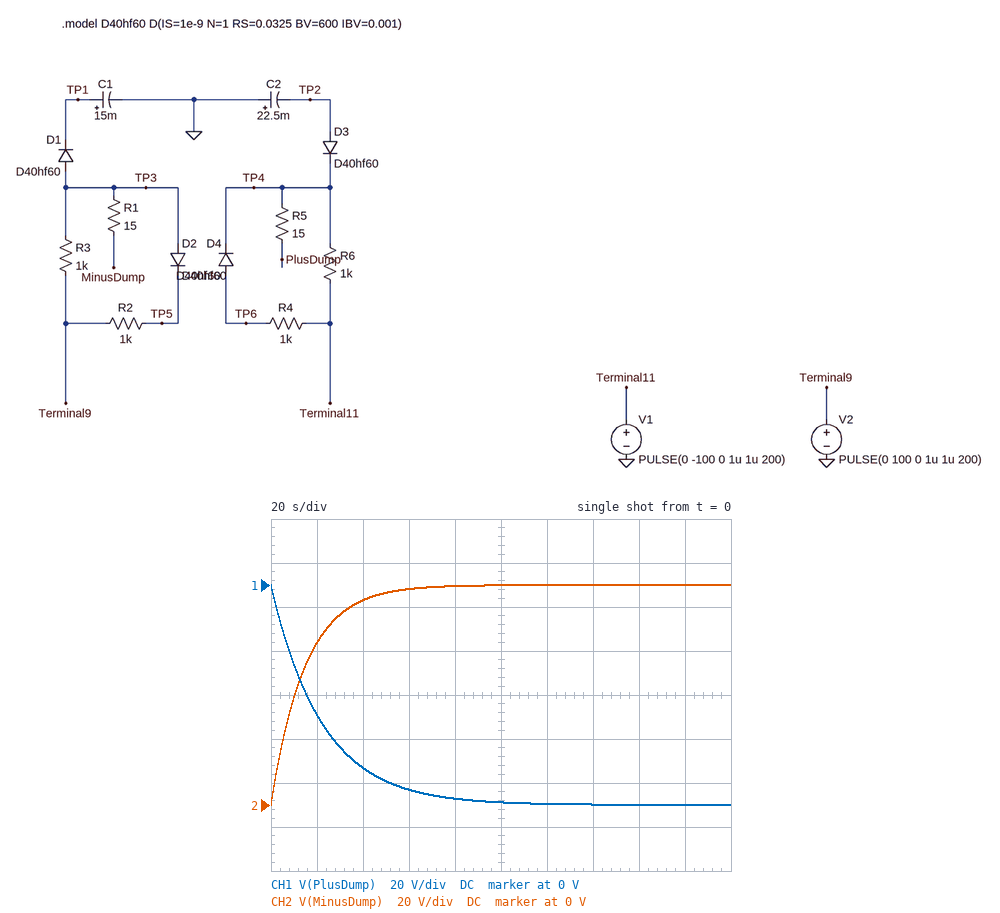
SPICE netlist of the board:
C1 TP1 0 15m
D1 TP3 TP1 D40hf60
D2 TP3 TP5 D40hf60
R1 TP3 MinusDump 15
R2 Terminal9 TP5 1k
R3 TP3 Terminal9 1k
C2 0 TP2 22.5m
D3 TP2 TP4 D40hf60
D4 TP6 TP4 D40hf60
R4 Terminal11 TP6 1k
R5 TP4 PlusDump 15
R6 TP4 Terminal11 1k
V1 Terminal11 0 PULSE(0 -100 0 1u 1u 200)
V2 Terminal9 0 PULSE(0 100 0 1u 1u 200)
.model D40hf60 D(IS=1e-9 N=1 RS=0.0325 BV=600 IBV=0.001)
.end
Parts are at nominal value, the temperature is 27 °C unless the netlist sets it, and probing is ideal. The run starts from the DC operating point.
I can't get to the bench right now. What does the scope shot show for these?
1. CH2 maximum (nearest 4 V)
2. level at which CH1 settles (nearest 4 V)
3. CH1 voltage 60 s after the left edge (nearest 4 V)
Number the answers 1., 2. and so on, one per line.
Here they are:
1. 100 V
2. -100 V
3. -92 V
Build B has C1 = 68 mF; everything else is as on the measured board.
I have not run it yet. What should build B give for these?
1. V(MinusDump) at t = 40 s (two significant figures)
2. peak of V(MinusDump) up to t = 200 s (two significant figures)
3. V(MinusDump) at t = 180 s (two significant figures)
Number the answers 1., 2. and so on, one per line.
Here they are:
1. 45 V
2. 95 V
3. 93 V
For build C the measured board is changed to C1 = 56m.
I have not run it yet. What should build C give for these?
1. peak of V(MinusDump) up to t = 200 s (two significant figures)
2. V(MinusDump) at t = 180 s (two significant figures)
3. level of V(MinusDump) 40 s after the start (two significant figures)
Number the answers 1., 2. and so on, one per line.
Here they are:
1. 97 V
2. 96 V
3. 51 V
